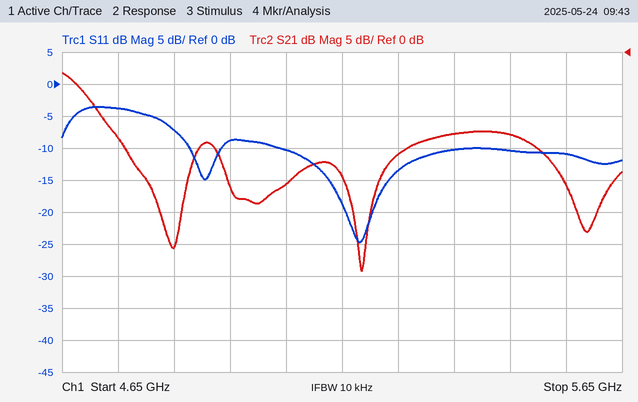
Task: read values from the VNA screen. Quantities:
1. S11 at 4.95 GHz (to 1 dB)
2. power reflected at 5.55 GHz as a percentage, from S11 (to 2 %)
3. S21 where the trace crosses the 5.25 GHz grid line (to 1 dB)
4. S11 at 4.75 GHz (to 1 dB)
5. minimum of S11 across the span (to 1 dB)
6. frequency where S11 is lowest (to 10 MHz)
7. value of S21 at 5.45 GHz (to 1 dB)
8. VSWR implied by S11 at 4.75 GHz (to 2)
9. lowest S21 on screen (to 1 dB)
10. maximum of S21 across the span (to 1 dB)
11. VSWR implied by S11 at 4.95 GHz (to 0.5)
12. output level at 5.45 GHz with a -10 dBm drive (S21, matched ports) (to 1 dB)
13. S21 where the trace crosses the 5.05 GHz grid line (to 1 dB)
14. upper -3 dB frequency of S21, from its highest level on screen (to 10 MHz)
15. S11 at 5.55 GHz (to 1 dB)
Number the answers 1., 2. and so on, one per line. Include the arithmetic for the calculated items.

1. -9 dB
2. 10^(-11/10) ≈ 8 %
3. -16 dB
4. -4 dB
5. -25 dB
6. 5.18 GHz
7. -13 dB
8. |Γ| = 10^(-4/20) = 0.6310; VSWR = (1 + 0.6310)/(1 − 0.6310) ≈ 4
9. -34 dB
10. -3 dB
11. |Γ| = 10^(-9/20) = 0.3548; VSWR = (1 + 0.3548)/(1 − 0.3548) ≈ 2.10, so 2.0 to the nearest 0.5
12. -10 dBm + (-13 dB) = -23 dBm
13. -21 dB
14. 4.69 GHz
15. -11 dB
